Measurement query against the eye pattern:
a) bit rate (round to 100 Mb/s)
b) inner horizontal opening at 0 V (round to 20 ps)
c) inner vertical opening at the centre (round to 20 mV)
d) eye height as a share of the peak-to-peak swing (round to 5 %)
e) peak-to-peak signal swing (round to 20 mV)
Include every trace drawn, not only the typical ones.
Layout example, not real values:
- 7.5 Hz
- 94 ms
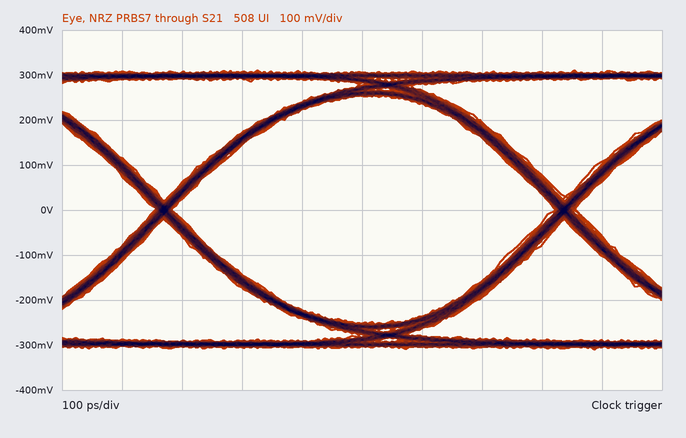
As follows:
- 1.5 Gb/s
- 640 ps
- 500 mV
- 80 %
- 620 mV
